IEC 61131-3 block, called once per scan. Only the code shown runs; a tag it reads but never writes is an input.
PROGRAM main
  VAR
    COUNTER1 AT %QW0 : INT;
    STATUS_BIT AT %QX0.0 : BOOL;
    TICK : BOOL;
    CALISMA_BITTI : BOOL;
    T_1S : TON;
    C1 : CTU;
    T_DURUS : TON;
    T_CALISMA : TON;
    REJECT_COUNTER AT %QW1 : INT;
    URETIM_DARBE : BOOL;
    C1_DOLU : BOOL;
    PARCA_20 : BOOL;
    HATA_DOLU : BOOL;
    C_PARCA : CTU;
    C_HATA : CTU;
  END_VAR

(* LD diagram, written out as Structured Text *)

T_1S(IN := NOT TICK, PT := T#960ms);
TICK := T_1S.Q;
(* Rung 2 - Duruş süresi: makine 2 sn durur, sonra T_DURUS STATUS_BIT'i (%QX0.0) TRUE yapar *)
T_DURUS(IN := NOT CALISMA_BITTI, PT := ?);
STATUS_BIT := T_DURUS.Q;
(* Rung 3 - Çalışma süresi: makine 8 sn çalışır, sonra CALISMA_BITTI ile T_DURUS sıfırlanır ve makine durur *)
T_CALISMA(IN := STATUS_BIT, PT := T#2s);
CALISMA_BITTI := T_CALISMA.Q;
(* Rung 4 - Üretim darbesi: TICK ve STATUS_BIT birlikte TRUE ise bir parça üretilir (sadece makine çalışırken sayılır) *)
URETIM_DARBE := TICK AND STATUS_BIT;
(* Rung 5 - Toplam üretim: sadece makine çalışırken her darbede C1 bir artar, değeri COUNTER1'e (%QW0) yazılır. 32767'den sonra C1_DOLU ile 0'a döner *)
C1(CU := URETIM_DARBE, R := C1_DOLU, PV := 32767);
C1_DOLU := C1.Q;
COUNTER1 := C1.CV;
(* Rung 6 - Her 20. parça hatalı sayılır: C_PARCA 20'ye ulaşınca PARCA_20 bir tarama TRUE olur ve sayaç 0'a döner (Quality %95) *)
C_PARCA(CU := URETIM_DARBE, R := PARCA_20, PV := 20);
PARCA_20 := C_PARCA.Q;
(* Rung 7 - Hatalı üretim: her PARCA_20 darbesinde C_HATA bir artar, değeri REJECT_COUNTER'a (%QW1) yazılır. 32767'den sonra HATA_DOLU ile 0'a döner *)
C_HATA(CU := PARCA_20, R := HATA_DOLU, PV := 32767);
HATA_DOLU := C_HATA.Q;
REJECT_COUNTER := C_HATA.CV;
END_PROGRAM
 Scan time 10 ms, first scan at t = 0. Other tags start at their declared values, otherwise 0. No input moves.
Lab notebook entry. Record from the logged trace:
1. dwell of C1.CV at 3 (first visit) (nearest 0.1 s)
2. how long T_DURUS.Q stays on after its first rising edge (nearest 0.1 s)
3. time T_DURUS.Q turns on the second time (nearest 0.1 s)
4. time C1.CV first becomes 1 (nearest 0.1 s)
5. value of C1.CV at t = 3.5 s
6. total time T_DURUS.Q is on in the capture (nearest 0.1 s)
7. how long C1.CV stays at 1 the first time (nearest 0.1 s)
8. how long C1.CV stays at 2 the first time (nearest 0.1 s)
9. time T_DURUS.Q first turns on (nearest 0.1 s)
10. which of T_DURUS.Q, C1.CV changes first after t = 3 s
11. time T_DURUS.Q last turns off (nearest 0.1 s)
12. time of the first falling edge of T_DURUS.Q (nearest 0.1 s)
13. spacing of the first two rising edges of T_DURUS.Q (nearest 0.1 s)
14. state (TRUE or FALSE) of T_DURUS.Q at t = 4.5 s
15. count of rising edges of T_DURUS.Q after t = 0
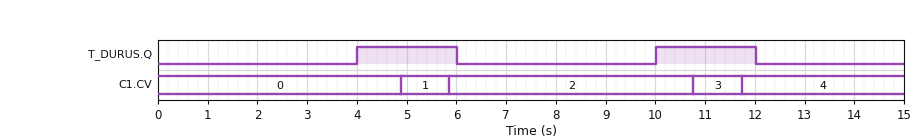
1.0 s
2.0 s
10.0 s
4.9 s
0
4.0 s
1.0 s
4.9 s
4.0 s
T_DURUS.Q
12.0 s
6.0 s
6.0 s
TRUE
2
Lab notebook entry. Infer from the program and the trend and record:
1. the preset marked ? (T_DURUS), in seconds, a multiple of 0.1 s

4.0 s
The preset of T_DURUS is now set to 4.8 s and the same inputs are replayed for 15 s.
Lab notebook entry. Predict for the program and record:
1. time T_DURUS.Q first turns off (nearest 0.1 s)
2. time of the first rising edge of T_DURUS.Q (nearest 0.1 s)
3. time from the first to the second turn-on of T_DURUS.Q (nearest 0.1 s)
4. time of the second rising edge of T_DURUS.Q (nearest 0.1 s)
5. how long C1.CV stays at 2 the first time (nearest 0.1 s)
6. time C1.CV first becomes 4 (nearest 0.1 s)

6.8 s
4.8 s
6.8 s
11.6 s
5.9 s
12.7 s
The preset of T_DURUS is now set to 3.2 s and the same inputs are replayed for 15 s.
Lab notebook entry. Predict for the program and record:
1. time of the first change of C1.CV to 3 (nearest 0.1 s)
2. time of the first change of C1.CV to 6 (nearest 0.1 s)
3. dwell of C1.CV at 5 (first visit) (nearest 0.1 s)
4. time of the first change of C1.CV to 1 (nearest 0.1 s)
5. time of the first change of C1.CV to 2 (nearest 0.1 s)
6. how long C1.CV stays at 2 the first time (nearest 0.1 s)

8.8 s
14.7 s
1.0 s
3.9 s
4.9 s
3.9 s
